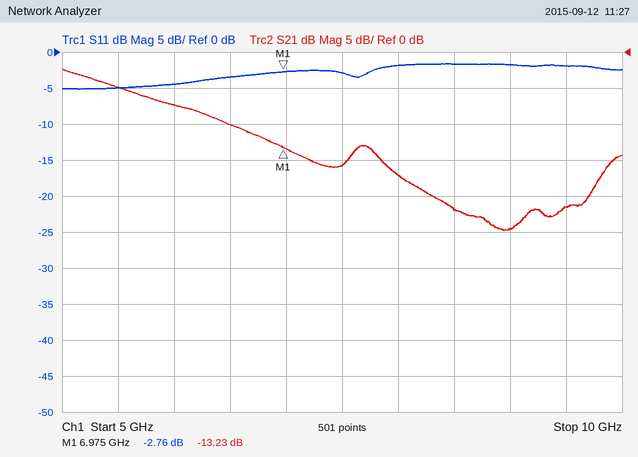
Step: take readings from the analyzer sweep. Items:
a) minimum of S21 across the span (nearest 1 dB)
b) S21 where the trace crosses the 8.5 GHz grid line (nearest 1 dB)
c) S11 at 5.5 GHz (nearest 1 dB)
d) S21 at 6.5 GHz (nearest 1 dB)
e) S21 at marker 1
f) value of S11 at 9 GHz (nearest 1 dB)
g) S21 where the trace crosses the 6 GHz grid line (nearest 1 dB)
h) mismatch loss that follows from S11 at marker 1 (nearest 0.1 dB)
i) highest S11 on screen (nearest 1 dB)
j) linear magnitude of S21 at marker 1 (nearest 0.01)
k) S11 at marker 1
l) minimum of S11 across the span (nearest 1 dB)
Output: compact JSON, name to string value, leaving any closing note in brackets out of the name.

{"minimum of S21 across the span": "-25 dB", "S21 where the trace crosses the 8.5 GHz grid line": "-22 dB", "S11 at 5.5 GHz": "-5 dB", "S21 at 6.5 GHz": "-10 dB", "S21 at marker 1": "-13.23 dB", "value of S11 at 9 GHz": "-2 dB", "S21 where the trace crosses the 6 GHz grid line": "-7 dB", "mismatch loss that follows from S11 at marker 1": "3.3 dB", "highest S11 on screen": "-2 dB", "linear magnitude of S21 at marker 1": "0.22", "S11 at marker 1": "-2.76 dB", "minimum of S11 across the span": "-5 dB"}
